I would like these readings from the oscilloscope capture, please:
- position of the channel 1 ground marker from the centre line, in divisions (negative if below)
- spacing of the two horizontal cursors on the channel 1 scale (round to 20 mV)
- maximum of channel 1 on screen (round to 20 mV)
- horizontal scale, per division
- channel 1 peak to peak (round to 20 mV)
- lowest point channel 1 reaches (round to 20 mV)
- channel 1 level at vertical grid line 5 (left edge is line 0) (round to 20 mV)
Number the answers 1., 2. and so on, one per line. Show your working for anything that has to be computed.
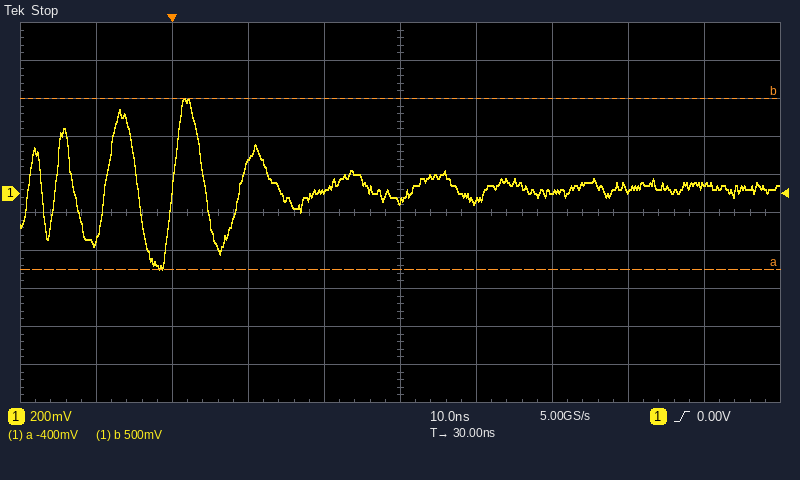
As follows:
1. +0.5 div
2. 900 mV
3. 500 mV
4. 10 ns
5. 500 mV − (-400 mV) = 900 mV
6. -400 mV
7. -40 mV
